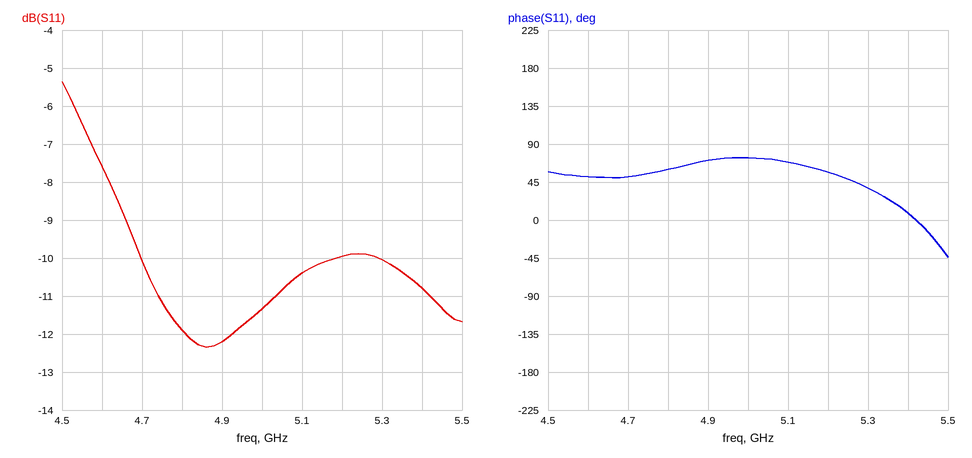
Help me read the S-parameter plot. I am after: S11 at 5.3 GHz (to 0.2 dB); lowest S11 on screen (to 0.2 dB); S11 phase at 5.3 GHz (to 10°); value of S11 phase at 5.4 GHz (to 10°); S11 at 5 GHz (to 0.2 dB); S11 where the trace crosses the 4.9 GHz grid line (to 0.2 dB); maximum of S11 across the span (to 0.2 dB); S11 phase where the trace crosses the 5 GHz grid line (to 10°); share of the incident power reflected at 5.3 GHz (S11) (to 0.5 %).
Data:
-10.0 dB
-12.4 dB
40°
10°
-11.4 dB
-12.2 dB
-5.4 dB
70°
10.0 %
